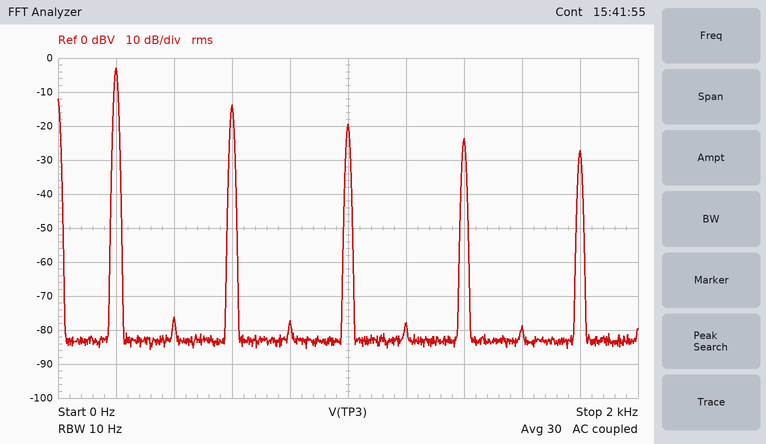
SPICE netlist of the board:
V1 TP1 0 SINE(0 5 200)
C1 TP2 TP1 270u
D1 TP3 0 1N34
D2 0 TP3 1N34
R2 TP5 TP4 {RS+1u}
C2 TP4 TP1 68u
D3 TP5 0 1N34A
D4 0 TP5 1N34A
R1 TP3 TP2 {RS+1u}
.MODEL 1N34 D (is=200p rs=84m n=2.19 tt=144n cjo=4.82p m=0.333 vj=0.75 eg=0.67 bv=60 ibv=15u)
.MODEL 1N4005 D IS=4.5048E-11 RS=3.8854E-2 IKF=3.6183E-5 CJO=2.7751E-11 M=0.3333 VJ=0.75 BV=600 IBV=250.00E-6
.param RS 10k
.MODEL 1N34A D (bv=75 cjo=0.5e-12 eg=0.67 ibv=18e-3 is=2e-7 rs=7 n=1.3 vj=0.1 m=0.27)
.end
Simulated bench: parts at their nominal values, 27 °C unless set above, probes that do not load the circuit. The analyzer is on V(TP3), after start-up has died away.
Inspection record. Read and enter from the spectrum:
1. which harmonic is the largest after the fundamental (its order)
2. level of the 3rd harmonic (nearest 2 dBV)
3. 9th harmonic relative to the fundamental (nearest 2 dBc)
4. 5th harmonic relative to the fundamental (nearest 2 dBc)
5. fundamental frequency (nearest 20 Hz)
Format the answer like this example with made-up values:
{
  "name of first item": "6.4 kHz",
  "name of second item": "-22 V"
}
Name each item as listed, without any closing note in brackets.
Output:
{
  "which harmonic is the largest after the fundamental": "3",
  "level of the 3rd harmonic": "-14 dBV",
  "9th harmonic relative to the fundamental": "-24 dBc",
  "5th harmonic relative to the fundamental": "-16 dBc",
  "fundamental frequency": "200 Hz"
}
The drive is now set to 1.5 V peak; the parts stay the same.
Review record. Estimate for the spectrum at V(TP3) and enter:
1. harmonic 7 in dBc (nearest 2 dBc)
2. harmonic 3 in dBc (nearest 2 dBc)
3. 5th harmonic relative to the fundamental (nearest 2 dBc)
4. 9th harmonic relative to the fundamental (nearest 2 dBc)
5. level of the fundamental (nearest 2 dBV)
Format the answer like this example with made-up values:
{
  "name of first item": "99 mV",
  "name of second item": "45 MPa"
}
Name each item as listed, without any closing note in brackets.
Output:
{
  "harmonic 7 in dBc": "-44 dBc",
  "harmonic 3 in dBc": "-14 dBc",
  "5th harmonic relative to the fundamental": "-26 dBc",
  "9th harmonic relative to the fundamental": "-44 dBc",
  "level of the fundamental": "-4 dBV"
}
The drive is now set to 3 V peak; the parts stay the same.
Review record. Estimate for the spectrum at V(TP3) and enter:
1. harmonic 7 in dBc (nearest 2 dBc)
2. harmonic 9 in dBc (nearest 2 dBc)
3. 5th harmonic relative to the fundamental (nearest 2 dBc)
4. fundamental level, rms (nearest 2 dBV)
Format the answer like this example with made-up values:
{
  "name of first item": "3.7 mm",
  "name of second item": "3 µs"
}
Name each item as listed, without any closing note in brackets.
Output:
{
  "harmonic 7 in dBc": "-24 dBc",
  "harmonic 9 in dBc": "-30 dBc",
  "5th harmonic relative to the fundamental": "-18 dBc",
  "fundamental level, rms": "-4 dBV"
}
